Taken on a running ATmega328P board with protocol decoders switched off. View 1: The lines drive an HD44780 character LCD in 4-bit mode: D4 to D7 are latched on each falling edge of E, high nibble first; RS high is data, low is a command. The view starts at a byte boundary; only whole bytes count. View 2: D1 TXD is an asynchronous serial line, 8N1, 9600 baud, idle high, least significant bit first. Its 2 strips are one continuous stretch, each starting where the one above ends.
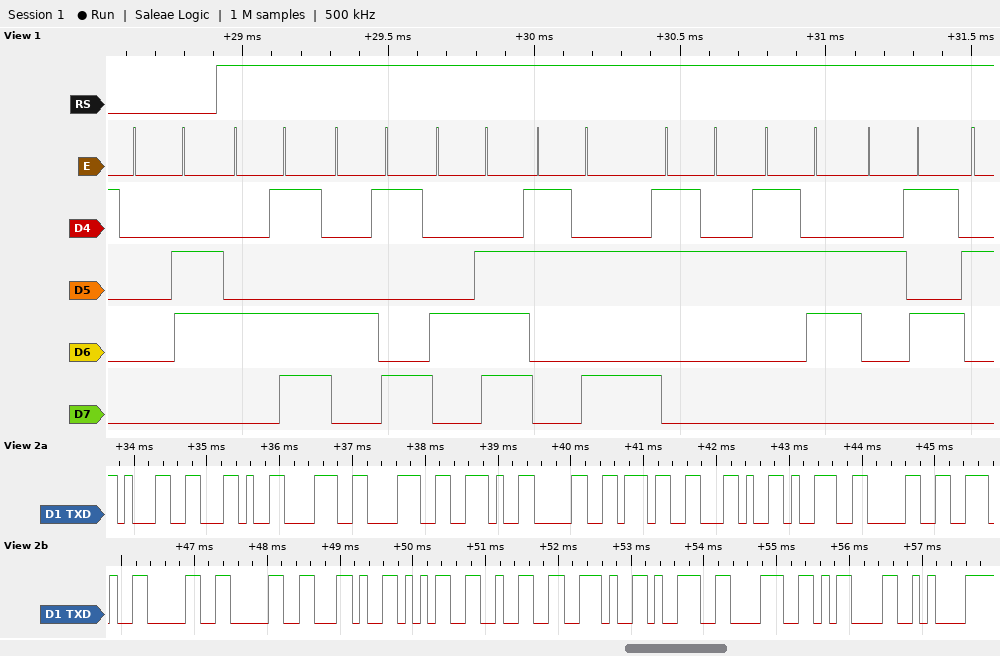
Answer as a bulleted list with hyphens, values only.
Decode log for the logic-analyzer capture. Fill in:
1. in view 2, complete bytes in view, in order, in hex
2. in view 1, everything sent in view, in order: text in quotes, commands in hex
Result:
- 0x31 0x2C 0x38 0x38 0x2E 0x30 0x37 0x2C 0x39 0x30 0x2E 0x30 0x30 0x2C 0x35 0x32 0x2E 0x39 0x38 0x0D 0x0A
- 0x06 "MIN:26%"
